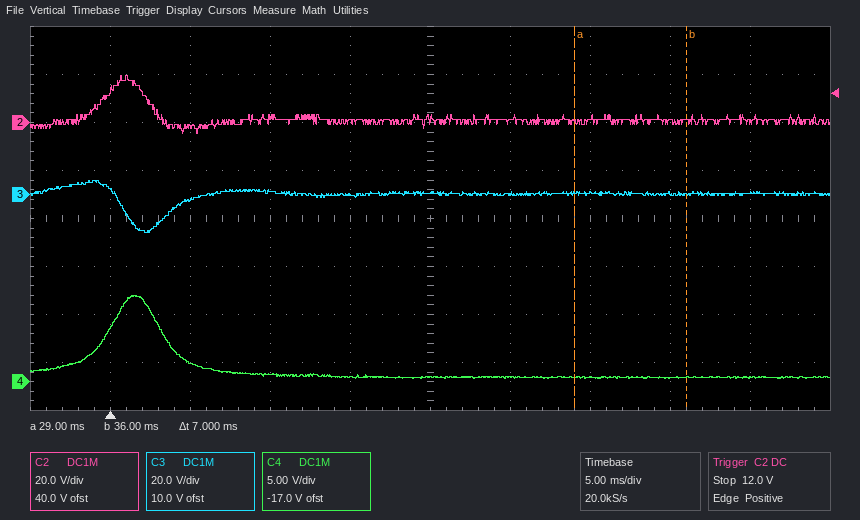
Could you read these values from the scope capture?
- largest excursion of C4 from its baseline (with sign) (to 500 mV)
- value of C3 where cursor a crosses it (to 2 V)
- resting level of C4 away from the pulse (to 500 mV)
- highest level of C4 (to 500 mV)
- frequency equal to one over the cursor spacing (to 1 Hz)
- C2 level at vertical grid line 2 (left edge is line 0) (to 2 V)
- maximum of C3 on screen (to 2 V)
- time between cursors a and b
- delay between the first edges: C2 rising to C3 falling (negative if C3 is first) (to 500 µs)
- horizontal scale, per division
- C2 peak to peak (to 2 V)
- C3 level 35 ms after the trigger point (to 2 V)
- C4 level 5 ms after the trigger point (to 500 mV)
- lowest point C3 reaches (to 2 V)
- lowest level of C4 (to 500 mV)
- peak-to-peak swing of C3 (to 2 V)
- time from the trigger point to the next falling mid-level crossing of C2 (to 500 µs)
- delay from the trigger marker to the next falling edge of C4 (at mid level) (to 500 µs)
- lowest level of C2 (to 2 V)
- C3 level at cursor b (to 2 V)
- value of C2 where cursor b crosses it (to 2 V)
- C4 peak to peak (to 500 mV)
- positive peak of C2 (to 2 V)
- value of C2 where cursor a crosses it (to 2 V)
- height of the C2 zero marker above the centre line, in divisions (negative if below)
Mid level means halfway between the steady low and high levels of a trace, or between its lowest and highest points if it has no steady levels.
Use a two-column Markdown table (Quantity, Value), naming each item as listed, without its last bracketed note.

| Quantity | Value |
|---|---|
| largest excursion of C4 from its baseline (with sign) | +8.5 V |
| value of C3 where cursor a crosses it | 0 V |
| resting level of C4 away from the pulse | 500 mV |
| highest level of C4 | 9.0 V |
| frequency equal to one over the cursor spacing | 143 Hz |
| C2 level at vertical grid line 2 (left edge is line 0) | -2 V |
| maximum of C3 on screen | 6 V |
| time between cursors a and b | 7 ms |
| delay between the first edges: C2 rising to C3 falling (negative if C3 is first) | +1.5 ms |
| horizontal scale, per division | 5 ms |
| C2 peak to peak | 24 V |
| C3 level 35 ms after the trigger point | 0 V |
| C4 level 5 ms after the trigger point | 2.0 V |
| lowest point C3 reaches | -16 V |
| lowest level of C4 | 500 mV |
| peak-to-peak swing of C3 | 22 V |
| time from the trigger point to the next falling mid-level crossing of C2 | 2.5 ms |
| delay from the trigger marker to the next falling edge of C4 (at mid level) | 3.5 ms |
| lowest level of C2 | -4 V |
| C3 level at cursor b | 0 V |
| value of C2 where cursor b crosses it | 0 V |
| C4 peak to peak | 8.5 V |
| positive peak of C2 | 20 V |
| value of C2 where cursor a crosses it | 0 V |
| height of the C2 zero marker above the centre line, in divisions | +2.0 div |
